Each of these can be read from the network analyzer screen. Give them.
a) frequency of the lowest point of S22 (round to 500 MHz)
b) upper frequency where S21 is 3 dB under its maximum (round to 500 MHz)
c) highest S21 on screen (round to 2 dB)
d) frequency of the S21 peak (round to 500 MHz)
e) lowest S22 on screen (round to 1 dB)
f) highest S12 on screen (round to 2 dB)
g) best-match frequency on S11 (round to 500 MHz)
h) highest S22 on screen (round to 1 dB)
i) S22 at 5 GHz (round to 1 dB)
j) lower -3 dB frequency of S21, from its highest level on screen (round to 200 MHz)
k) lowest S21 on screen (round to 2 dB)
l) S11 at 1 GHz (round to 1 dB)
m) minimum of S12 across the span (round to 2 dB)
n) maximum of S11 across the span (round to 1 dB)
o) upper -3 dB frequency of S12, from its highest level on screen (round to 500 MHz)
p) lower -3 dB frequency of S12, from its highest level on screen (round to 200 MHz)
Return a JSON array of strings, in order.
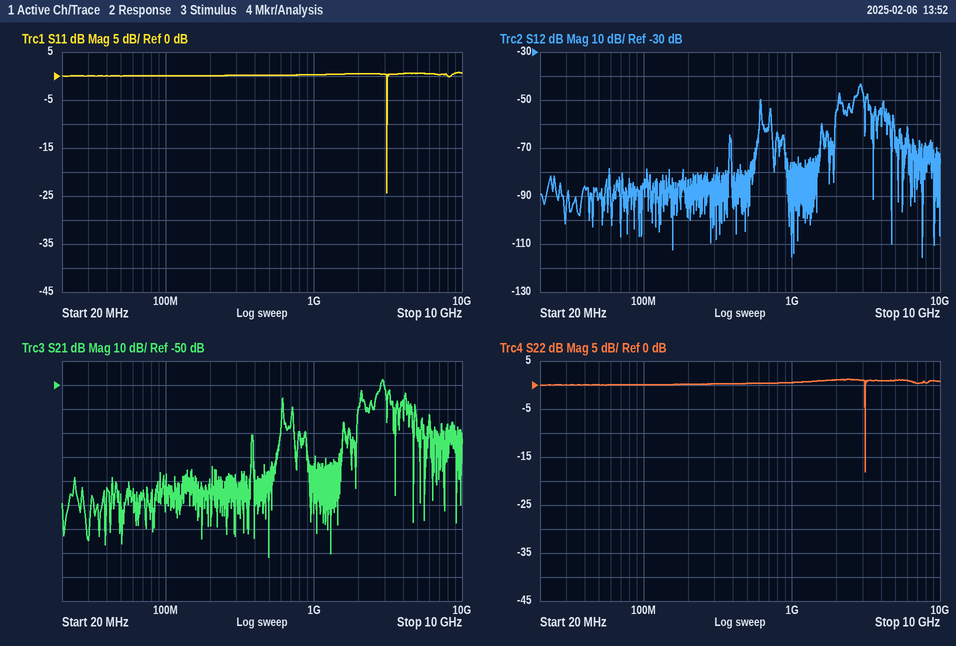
["3.0 GHz", "3.0 GHz", "-48 dB", "3.0 GHz", "-18 dB", "-44 dB", "3.0 GHz", "1 dB", "1 dB", "2.8 GHz", "-122 dB", "0 dB", "-116 dB", "1 dB", "3.0 GHz", "2.8 GHz"]
